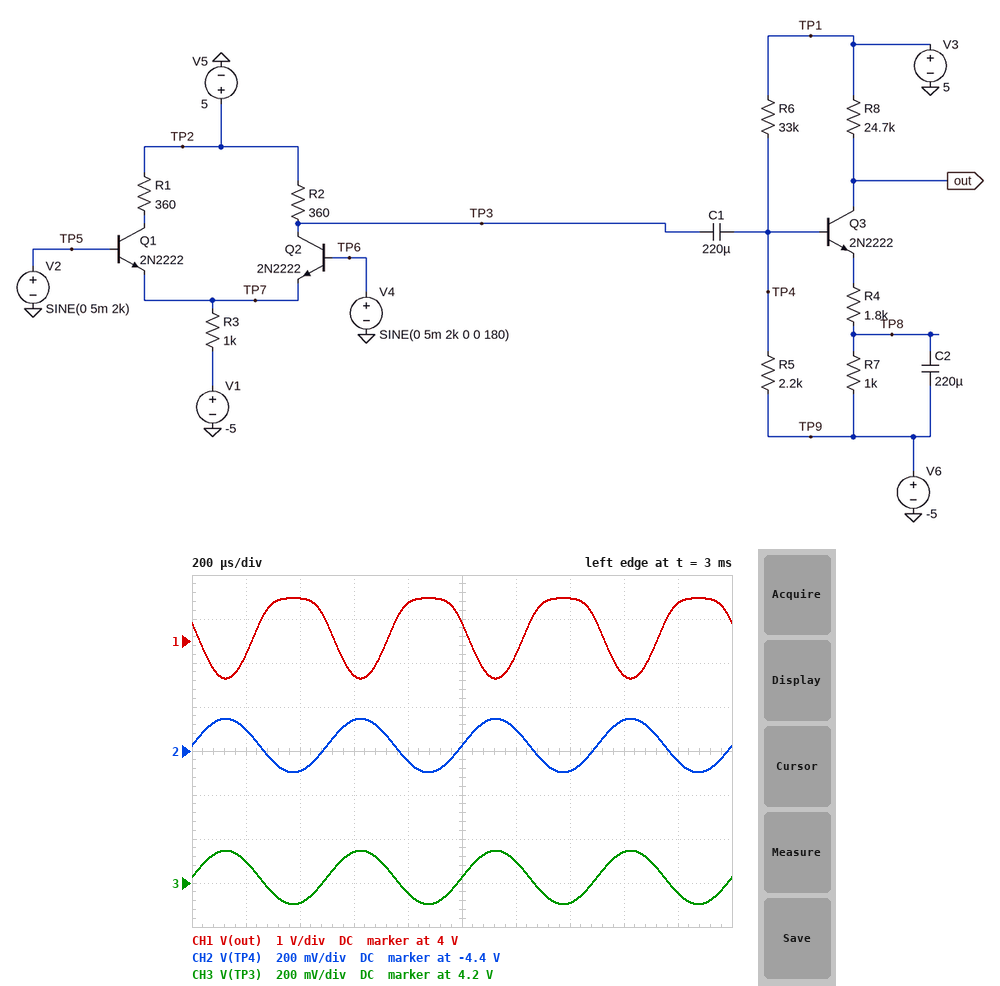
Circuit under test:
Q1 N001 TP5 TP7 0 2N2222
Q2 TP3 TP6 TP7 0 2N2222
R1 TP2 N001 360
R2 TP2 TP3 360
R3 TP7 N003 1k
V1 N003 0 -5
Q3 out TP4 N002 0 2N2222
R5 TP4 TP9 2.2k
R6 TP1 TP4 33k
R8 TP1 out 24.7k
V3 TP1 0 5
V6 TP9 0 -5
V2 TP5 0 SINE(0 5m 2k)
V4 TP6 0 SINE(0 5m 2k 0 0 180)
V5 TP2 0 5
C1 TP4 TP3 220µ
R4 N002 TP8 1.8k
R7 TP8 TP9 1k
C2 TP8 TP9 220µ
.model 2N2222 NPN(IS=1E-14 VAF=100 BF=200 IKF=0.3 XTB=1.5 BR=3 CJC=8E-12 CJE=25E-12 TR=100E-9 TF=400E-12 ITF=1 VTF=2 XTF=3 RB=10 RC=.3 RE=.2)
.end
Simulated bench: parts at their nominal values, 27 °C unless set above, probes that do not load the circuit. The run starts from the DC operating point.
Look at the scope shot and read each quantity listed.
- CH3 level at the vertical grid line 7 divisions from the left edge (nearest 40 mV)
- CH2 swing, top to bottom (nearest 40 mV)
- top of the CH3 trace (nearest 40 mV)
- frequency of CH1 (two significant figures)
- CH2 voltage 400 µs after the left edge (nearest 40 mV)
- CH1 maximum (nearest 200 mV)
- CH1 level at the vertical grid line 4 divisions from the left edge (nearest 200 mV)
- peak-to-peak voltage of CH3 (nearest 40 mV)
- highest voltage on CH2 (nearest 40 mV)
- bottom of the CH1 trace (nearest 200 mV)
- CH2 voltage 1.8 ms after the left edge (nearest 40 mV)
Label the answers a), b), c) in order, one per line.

a) 4.12 V
b) 240 mV
c) 4.36 V
d) 2.0 kHz
e) -4.48 V
f) 5.0 V
g) 4.8 V
h) 240 mV
i) -4.24 V
j) 3.2 V
k) -4.44 V
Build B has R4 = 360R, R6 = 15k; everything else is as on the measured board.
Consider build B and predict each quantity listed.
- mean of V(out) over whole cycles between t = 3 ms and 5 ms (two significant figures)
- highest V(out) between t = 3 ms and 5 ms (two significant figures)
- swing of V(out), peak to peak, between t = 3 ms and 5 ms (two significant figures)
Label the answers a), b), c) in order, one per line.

a) -3.1 V
b) 320 mV
c) 4.7 V
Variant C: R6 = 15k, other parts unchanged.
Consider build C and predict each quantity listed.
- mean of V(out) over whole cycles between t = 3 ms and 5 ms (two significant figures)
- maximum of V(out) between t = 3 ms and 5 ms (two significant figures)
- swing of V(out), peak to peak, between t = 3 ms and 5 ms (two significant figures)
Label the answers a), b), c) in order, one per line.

a) -800 mV
b) 740 mV
c) 3.1 V
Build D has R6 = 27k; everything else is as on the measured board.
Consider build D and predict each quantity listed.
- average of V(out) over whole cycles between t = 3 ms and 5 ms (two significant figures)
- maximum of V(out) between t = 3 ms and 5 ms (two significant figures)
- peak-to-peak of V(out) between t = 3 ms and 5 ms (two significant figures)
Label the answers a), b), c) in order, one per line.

a) 3.4 V
b) 4.6 V
c) 2.6 V
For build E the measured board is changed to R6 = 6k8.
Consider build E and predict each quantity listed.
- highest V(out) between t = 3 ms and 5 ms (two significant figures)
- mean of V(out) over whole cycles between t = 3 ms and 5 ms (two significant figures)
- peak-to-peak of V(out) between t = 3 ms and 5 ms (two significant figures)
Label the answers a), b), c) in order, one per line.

a) -3.4 V
b) -3.5 V
c) 180 mV
